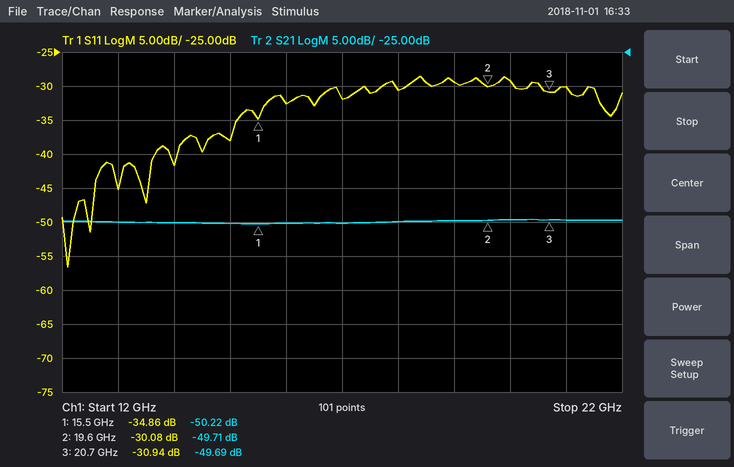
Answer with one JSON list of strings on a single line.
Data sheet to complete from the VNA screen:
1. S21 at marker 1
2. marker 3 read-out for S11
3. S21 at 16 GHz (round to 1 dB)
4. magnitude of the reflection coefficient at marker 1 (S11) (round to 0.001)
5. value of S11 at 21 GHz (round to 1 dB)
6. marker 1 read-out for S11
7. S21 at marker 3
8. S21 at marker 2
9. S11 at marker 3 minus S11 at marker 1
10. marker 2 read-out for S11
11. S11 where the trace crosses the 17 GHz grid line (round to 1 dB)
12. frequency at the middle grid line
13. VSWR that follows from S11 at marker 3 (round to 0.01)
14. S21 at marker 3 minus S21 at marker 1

["-50.22 dB", "-30.94 dB", "-50 dB", "0.018", "-30 dB", "-34.86 dB", "-49.69 dB", "-49.71 dB", "3.92 dB", "-30.08 dB", "-32 dB", "17 GHz", "1.06", "0.53 dB"]
